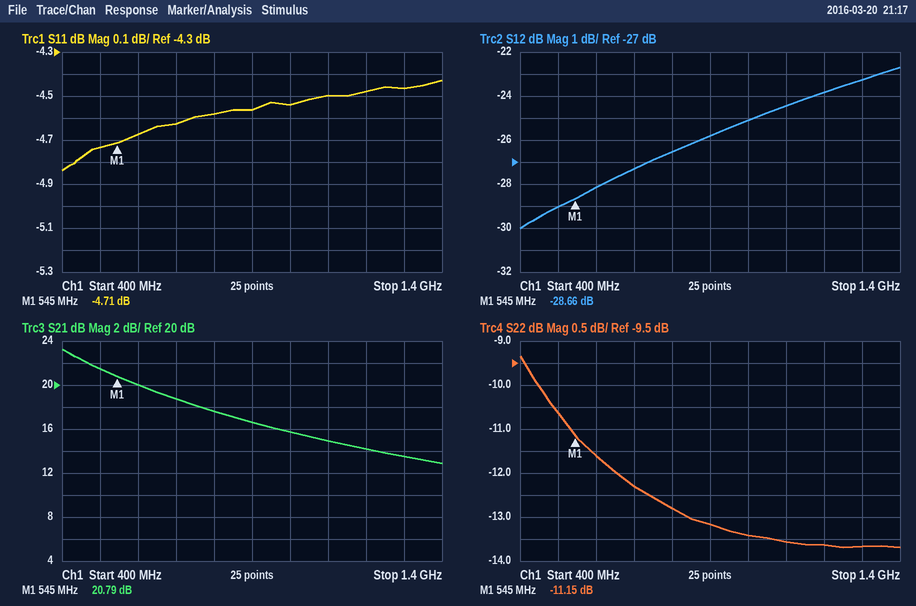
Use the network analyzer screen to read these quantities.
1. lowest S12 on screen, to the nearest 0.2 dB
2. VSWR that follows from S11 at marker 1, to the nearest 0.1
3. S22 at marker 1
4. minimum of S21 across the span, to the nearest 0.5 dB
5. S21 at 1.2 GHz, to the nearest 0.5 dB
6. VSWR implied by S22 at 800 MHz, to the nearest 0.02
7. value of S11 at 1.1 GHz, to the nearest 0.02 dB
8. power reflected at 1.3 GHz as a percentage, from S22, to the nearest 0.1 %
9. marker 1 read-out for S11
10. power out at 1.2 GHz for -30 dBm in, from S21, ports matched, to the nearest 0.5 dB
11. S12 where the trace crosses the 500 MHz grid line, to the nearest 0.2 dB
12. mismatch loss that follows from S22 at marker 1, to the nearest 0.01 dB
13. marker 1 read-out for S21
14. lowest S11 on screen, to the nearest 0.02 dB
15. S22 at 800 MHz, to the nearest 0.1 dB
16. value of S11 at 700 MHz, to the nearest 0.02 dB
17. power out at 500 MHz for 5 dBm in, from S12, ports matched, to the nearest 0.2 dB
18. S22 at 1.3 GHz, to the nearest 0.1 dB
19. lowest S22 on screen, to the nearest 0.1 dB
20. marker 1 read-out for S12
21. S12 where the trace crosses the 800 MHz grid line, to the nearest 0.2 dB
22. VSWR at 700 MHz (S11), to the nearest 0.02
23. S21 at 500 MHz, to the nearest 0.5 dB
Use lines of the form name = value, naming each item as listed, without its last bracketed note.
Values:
lowest S12 on screen, to the nearest 0.2 dB = -30.0 dB
VSWR that follows from S11 at marker 1, to the nearest 0.1 = 3.8
S22 at marker 1 = -11.15 dB
minimum of S21 across the span, to the nearest 0.5 dB = 13.0 dB
S21 at 1.2 GHz, to the nearest 0.5 dB = 14.0 dB
VSWR implied by S22 at 800 MHz, to the nearest 0.02 = 1.60
value of S11 at 1.1 GHz, to the nearest 0.02 dB = -4.50 dB
power reflected at 1.3 GHz as a percentage, from S22, to the nearest 0.1 % = 4.3 %
marker 1 read-out for S11 = -4.71 dB
power out at 1.2 GHz for -30 dBm in, from S21, ports matched, to the nearest 0.5 dB = -16.0 dBm
S12 where the trace crosses the 500 MHz grid line, to the nearest 0.2 dB = -29.0 dB
mismatch loss that follows from S22 at marker 1, to the nearest 0.01 dB = 0.35 dB
marker 1 read-out for S21 = 20.79 dB
lowest S11 on screen, to the nearest 0.02 dB = -4.84 dB
S22 at 800 MHz, to the nearest 0.1 dB = -12.8 dB
value of S11 at 700 MHz, to the nearest 0.02 dB = -4.62 dB
power out at 500 MHz for 5 dBm in, from S12, ports matched, to the nearest 0.2 dB = -24.0 dBm
S22 at 1.3 GHz, to the nearest 0.1 dB = -13.7 dB
lowest S22 on screen, to the nearest 0.1 dB = -13.7 dB
marker 1 read-out for S12 = -28.66 dB
S12 where the trace crosses the 800 MHz grid line, to the nearest 0.2 dB = -26.6 dB
VSWR at 700 MHz (S11), to the nearest 0.02 = 3.84
S21 at 500 MHz, to the nearest 0.5 dB = 21.5 dB
